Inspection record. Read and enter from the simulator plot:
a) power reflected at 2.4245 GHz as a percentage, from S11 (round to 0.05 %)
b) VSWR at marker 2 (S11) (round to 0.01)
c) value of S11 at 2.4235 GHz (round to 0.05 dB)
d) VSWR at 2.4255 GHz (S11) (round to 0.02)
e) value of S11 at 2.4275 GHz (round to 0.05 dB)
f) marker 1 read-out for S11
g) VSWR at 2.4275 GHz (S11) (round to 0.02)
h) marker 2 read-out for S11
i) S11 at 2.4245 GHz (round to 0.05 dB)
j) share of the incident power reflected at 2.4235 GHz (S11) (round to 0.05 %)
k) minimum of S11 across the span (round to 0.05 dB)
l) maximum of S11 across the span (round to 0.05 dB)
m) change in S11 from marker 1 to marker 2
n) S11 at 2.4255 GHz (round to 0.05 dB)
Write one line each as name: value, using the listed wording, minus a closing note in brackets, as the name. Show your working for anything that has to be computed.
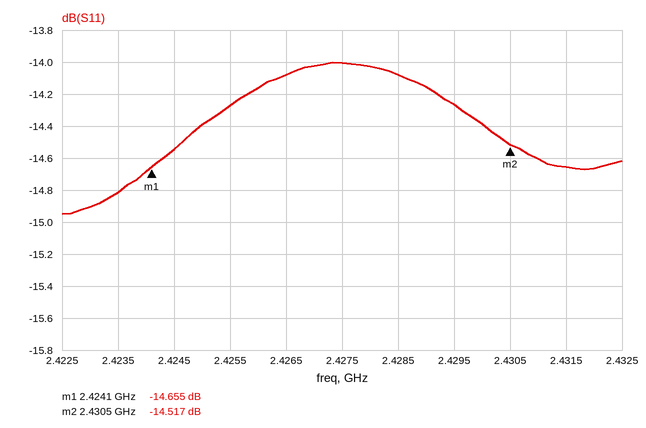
power reflected at 2.4245 GHz as a percentage, from S11: 10^(-14.55/10) ≈ 3.51 %, so 3.50 % to the nearest 0.05 %
VSWR at marker 2 (S11): (1 + 0.1880)/(1 − 0.1880) ≈ 1.46
value of S11 at 2.4235 GHz: -14.80 dB
VSWR at 2.4255 GHz (S11): |Γ| = 10^(-14.25/20) = 0.1939; VSWR = (1 + 0.1939)/(1 − 0.1939) ≈ 1.48
value of S11 at 2.4275 GHz: -14.00 dB
marker 1 read-out for S11: -14.655 dB
VSWR at 2.4275 GHz (S11): |Γ| = 10^(-14/20) = 0.1995; VSWR = (1 + 0.1995)/(1 − 0.1995) ≈ 1.50
marker 2 read-out for S11: -14.517 dB
S11 at 2.4245 GHz: -14.55 dB
share of the incident power reflected at 2.4235 GHz (S11): 10^(-14.8/10) ≈ 3.31 %, so 3.30 % to the nearest 0.05 %
minimum of S11 across the span: -14.95 dB
maximum of S11 across the span: -14.00 dB
change in S11 from marker 1 to marker 2: -14.517 − (-14.655) = 0.138 dB
S11 at 2.4255 GHz: -14.25 dB
